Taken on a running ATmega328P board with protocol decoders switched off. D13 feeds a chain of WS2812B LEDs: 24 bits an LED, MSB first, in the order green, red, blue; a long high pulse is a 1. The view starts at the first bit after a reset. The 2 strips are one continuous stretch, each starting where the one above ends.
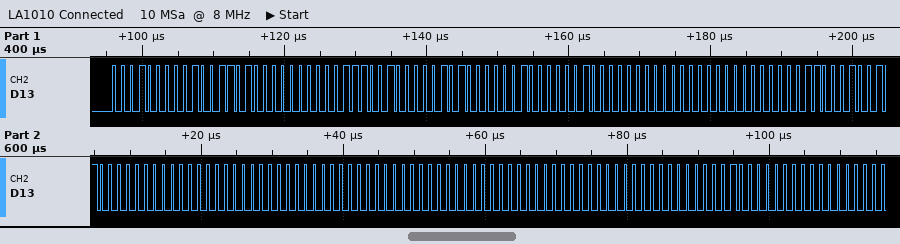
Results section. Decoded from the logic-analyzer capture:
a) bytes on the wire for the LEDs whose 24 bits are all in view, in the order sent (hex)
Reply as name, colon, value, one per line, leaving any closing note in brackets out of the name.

bytes on the wire for the LEDs whose 24 bits are all in view, in the order sent: 10 4D 00 39 05 02 04 00 00 03 13 00 00 00 00 00 00 00 00 01 00
